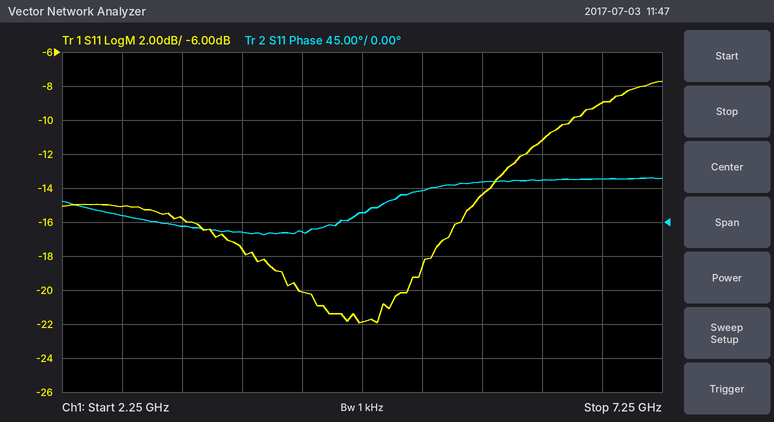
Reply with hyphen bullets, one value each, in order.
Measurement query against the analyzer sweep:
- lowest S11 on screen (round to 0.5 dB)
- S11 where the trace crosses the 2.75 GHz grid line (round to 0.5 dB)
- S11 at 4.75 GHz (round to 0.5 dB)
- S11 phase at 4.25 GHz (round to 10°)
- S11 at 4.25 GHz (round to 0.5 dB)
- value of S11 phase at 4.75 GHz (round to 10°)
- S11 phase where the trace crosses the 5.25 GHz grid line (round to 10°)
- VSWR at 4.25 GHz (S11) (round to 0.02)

- -22.0 dB
- -15.0 dB
- -22.0 dB
- -10°
- -20.0 dB
- 10°
- 40°
- 1.22
